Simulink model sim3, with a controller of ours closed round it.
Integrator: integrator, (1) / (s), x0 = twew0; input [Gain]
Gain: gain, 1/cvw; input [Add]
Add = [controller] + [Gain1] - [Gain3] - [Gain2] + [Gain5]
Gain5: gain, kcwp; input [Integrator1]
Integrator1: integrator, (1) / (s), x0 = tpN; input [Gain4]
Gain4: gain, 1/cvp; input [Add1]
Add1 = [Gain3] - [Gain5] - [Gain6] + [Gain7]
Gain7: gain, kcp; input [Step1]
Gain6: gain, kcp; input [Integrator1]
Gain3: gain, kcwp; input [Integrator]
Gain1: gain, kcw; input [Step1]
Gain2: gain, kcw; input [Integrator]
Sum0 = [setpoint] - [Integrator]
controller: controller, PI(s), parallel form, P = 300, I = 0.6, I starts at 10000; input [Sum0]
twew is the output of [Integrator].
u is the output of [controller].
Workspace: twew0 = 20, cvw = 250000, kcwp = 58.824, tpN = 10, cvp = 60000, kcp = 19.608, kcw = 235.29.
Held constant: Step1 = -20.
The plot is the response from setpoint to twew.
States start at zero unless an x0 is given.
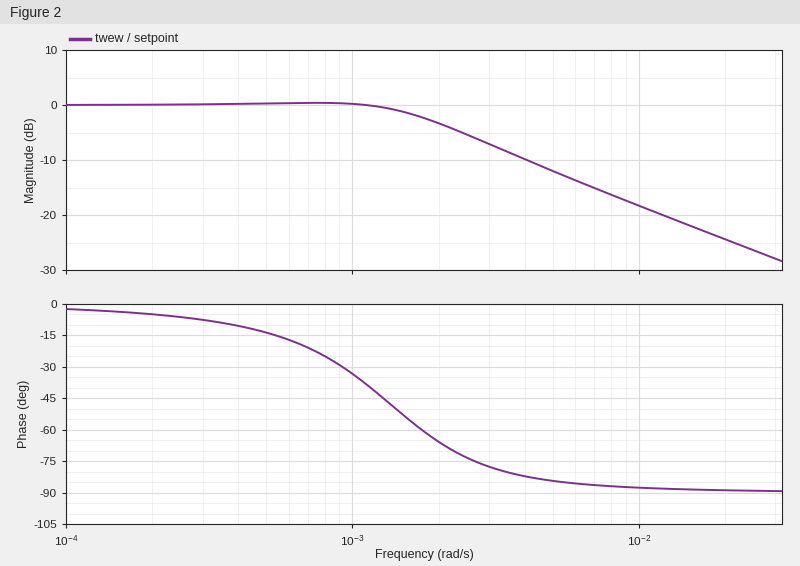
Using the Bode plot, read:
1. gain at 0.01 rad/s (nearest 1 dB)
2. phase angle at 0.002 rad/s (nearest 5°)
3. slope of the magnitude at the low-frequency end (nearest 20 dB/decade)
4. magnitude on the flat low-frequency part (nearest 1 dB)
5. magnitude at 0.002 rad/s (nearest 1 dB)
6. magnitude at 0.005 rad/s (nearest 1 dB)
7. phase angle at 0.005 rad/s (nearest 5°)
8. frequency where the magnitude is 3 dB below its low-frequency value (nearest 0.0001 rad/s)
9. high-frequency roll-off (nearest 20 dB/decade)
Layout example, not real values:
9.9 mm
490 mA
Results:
-18 dB
-65°
0 dB/decade
0 dB
-3 dB
-12 dB
-85°
0.0019 rad/s
-20 dB/decade
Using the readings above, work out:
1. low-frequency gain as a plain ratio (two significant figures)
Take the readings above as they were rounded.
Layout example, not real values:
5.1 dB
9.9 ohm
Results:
1.0
